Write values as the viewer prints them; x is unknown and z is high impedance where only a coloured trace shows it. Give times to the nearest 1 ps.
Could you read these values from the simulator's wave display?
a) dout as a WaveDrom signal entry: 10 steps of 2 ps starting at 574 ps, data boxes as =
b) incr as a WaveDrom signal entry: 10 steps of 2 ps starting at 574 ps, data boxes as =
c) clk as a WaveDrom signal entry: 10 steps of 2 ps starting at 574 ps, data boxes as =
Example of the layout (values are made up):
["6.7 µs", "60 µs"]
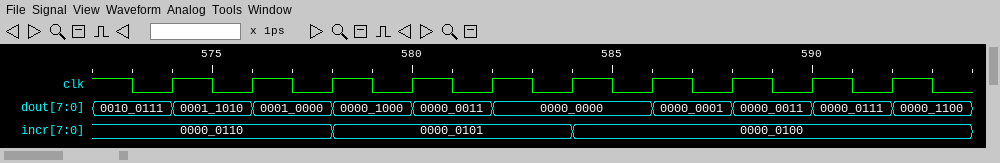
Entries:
["{name: 'dout', wave: '=====.====', data: '0001_1010 0001_0000 0000_1000 0000_0011 0000_0000 0000_0001 0000_0011 0000_0111 0000_1100'}", "{name: 'incr', wave: '=.=..=....', data: '0000_0110 0000_0101 0000_0100'}", "{name: 'clk', wave: 'p.........'}"]
